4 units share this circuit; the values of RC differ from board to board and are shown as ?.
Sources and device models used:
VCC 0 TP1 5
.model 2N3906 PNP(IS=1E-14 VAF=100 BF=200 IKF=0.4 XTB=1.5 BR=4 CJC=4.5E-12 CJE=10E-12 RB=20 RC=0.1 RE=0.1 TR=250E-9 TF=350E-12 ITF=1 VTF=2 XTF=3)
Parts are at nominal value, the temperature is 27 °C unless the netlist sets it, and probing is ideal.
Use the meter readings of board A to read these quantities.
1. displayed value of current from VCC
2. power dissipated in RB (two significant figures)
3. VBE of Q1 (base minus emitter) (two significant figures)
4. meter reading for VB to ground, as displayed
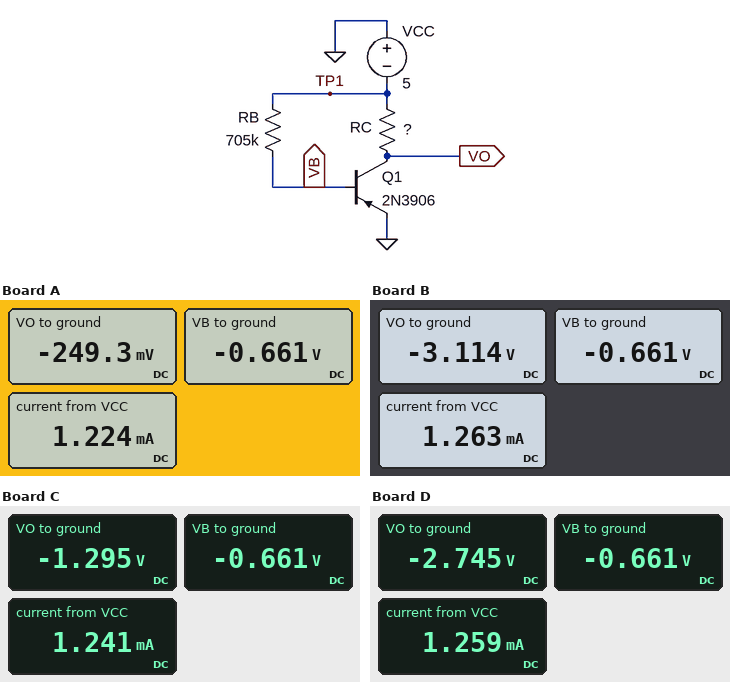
1.224 mA
27 µW
-660 mV
-0.661 V
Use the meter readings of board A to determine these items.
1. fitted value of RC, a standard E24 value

3.9 kΩ
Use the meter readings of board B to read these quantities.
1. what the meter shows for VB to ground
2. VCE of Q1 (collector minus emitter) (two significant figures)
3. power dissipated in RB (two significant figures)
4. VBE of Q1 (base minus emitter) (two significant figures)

-0.661 V
-3.1 V
27 µW
-660 mV
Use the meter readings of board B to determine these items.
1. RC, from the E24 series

1.5 kΩ
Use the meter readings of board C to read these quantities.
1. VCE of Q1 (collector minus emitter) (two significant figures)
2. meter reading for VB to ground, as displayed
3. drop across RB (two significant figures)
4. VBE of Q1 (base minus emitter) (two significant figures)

-1.3 V
-0.661 V
4.3 V
-660 mV
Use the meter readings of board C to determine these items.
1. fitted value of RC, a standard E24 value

3 kΩ
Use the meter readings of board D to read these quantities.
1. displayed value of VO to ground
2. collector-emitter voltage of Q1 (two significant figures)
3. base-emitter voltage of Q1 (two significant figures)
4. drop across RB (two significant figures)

-2.745 V
-2.7 V
-660 mV
4.3 V
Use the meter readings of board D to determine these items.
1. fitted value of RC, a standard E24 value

1.8 kΩ
